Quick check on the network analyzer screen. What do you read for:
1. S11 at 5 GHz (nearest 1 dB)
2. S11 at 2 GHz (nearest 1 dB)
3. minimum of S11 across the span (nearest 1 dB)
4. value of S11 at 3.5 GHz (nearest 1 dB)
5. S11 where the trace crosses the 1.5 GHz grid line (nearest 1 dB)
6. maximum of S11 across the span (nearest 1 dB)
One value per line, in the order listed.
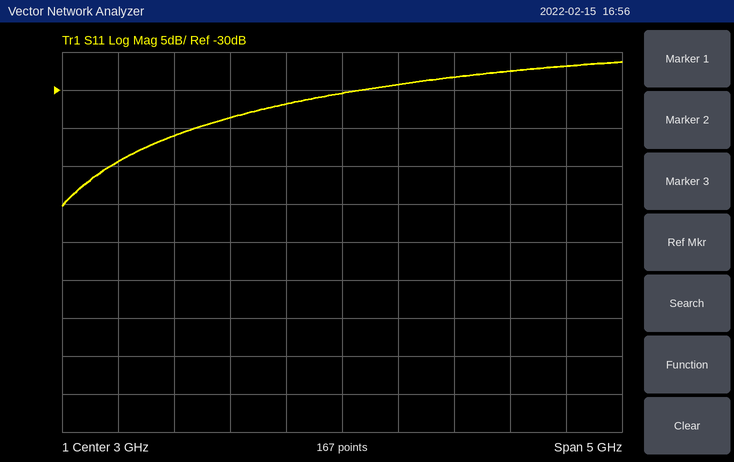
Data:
-27 dB
-34 dB
-45 dB
-29 dB
-36 dB
-26 dB
